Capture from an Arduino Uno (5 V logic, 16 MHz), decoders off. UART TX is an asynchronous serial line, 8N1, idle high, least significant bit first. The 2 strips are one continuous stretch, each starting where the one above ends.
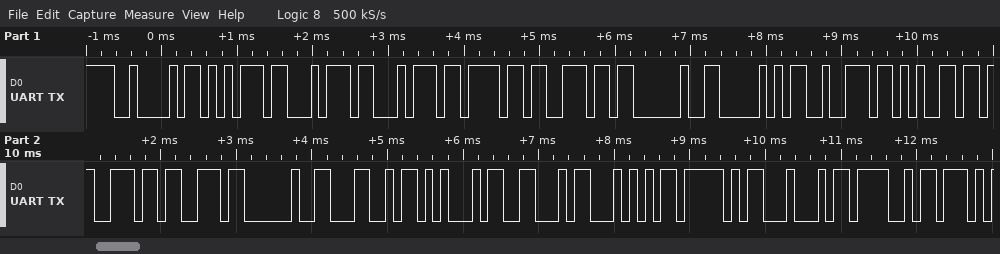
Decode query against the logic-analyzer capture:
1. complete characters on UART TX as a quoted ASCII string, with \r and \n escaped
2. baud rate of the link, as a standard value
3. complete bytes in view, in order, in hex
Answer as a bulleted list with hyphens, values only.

- "Button Press LEFT_DO"
- 9600 baud
- 0x42 0x75 0x74 0x74 0x6F 0x6E 0x20 0x50 0x72 0x65 0x73 0x73 0x20 0x4C 0x45 0x46 0x54 0x5F 0x44 0x4F
